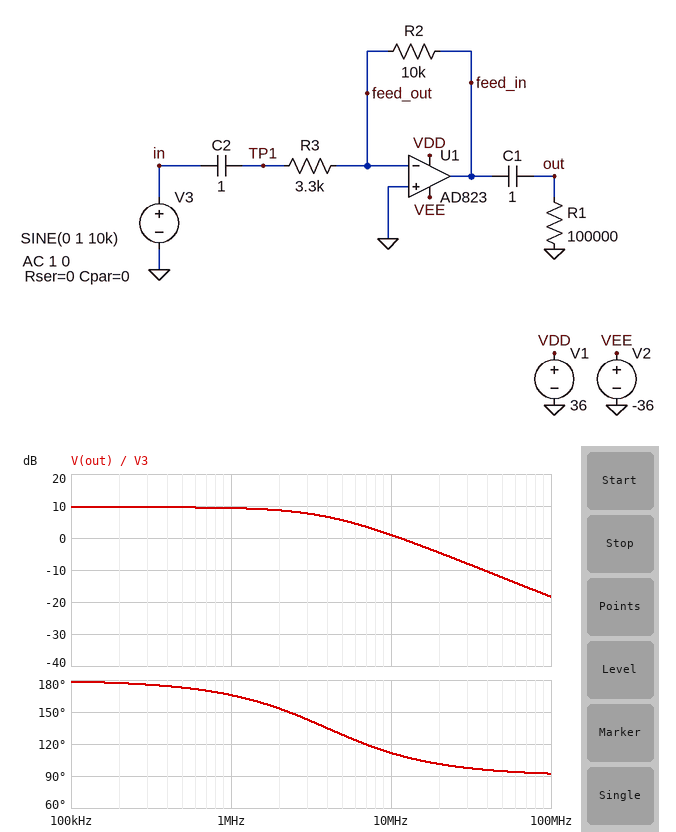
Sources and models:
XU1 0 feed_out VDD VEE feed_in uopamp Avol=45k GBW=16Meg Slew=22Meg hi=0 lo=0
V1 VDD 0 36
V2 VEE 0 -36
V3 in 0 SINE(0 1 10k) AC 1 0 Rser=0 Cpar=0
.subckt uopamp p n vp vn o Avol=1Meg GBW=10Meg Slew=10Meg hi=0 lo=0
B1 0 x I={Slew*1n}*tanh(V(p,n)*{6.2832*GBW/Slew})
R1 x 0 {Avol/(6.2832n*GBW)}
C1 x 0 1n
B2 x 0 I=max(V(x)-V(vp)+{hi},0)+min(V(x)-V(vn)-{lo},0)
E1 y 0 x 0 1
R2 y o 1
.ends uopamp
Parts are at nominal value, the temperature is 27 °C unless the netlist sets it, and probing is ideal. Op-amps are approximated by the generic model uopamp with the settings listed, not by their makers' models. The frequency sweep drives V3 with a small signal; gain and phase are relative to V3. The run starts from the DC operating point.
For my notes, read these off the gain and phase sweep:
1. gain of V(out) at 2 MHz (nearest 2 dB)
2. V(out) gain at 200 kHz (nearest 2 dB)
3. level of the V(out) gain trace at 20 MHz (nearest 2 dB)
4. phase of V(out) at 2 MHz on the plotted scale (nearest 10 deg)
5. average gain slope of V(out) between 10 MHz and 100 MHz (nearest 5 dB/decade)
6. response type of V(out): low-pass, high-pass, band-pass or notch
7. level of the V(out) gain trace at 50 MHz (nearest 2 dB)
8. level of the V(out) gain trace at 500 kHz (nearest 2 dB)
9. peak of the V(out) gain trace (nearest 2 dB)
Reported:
8 dB
10 dB
-4 dB
150 deg
-20 dB/decade
low-pass
-12 dB
10 dB
10 dB
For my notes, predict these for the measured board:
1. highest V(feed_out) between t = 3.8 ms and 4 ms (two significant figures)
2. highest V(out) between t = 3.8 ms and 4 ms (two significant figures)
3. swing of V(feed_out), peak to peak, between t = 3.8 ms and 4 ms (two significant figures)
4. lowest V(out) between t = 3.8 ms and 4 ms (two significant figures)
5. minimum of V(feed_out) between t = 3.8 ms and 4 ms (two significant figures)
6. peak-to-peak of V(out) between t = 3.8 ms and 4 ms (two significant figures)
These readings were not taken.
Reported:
1.9 mV
3.0 V
3.8 mV
-3.0 V
-1.9 mV
6.1 V
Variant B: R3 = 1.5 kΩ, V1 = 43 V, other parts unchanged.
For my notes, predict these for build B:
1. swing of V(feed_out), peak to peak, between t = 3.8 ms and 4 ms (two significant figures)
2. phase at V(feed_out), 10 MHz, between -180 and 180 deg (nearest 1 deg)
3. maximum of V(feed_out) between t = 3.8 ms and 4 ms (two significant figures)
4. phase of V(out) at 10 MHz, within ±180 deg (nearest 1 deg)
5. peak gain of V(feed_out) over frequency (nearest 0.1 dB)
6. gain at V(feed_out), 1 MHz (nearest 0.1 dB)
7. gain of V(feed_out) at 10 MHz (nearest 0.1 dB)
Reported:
8.3 mV
12 deg
4.2 mV
102 deg
-1.2 dB
-8.5 dB
-1.4 dB
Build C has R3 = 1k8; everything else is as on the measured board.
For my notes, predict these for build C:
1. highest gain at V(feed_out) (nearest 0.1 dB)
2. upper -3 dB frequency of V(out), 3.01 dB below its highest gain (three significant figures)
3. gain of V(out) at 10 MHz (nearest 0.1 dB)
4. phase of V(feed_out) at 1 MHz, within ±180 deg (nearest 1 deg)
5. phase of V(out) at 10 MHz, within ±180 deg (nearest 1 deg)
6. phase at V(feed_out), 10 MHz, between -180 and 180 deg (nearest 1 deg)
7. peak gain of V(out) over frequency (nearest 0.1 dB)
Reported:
-1.4 dB
2.44 MHz
2.4 dB
68 deg
104 deg
14 deg
14.9 dB
